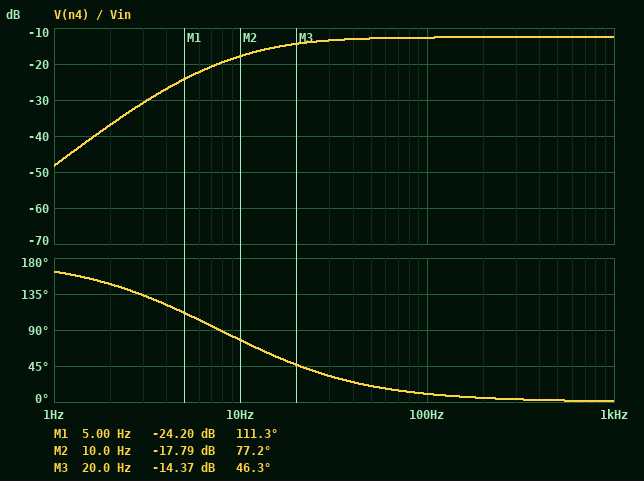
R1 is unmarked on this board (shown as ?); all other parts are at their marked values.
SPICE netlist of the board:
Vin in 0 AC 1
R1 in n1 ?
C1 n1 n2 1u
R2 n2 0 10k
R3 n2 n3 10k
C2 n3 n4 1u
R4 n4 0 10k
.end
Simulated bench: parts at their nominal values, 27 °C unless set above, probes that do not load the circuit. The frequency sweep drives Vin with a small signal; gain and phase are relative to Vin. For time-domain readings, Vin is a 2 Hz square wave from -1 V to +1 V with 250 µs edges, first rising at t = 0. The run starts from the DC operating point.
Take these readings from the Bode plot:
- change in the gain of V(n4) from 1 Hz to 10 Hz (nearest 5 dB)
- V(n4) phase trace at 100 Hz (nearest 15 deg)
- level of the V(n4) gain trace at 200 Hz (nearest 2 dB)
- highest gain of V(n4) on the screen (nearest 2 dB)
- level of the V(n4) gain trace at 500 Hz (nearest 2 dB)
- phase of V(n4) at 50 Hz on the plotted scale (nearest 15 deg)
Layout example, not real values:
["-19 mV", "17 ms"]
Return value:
["30 dB", "15 deg", "-12 dB", "-12 dB", "-12 dB", "15 deg"]
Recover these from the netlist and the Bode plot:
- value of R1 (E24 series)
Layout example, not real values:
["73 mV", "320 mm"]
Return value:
["7.5 kΩ"]
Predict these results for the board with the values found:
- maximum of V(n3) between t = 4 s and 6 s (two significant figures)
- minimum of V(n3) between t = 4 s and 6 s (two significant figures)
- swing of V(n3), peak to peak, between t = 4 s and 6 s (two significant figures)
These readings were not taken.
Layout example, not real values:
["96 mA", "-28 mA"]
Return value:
["470 mV", "-470 mV", "940 mV"]
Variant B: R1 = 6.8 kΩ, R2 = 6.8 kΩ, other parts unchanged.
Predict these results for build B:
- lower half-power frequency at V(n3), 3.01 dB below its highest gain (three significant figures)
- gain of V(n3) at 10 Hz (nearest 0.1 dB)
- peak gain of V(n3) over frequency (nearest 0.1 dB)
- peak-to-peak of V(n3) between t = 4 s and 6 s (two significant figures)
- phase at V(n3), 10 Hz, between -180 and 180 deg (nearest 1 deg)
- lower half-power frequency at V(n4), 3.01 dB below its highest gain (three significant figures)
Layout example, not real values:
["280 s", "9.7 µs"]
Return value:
["4.76 Hz", "-14.1 dB", "-13.4 dB", "850 mV", "26 deg", "16.5 Hz"]
